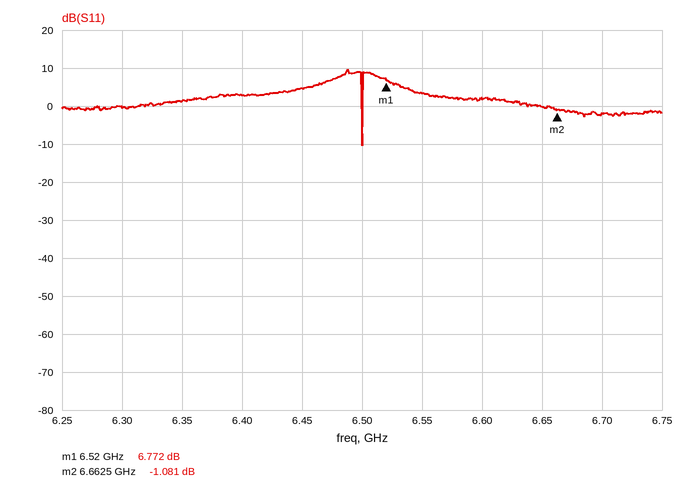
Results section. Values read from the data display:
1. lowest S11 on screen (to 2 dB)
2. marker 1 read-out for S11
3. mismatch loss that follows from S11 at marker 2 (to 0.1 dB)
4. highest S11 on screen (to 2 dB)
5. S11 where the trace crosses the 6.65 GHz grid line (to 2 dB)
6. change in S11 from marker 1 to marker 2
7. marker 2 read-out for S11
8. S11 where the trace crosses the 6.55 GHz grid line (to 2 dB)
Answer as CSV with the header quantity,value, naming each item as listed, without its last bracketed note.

quantity,value
lowest S11 on screen,-10 dB
marker 1 read-out for S11,6.772 dB
mismatch loss that follows from S11 at marker 2,6.6 dB
highest S11 on screen,10 dB
S11 where the trace crosses the 6.65 GHz grid line,0 dB
change in S11 from marker 1 to marker 2,-7.853 dB
marker 2 read-out for S11,-1.081 dB
S11 where the trace crosses the 6.55 GHz grid line,4 dB
